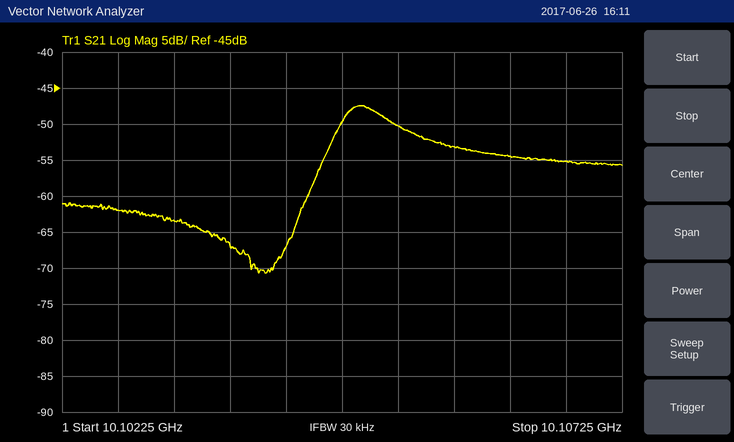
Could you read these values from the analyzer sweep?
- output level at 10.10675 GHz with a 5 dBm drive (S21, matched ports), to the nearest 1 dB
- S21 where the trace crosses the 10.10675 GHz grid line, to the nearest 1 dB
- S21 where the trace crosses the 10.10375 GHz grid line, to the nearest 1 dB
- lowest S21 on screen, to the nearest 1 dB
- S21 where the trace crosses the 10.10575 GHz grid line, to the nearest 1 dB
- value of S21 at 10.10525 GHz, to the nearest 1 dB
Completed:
-50 dBm
-55 dB
-67 dB
-71 dB
-53 dB
-50 dB
